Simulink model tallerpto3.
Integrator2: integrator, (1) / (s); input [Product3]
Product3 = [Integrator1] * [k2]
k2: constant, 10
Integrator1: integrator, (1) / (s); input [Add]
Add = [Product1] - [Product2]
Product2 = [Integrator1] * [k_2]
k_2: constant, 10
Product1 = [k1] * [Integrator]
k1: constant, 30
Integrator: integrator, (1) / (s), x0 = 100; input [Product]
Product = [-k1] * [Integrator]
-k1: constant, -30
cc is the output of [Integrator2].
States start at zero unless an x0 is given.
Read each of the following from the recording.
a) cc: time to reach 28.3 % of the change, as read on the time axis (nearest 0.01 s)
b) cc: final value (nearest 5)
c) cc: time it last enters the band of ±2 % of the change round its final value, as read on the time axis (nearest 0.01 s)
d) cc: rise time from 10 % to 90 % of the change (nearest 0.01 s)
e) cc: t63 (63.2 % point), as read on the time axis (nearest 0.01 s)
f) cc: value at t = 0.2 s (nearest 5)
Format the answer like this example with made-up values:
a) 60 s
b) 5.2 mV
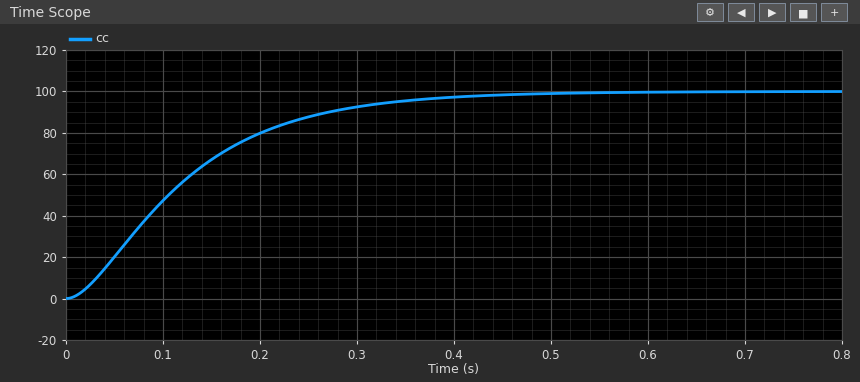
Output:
a) 0.06 s
b) 100
c) 0.43 s
d) 0.24 s
e) 0.14 s
f) 80
